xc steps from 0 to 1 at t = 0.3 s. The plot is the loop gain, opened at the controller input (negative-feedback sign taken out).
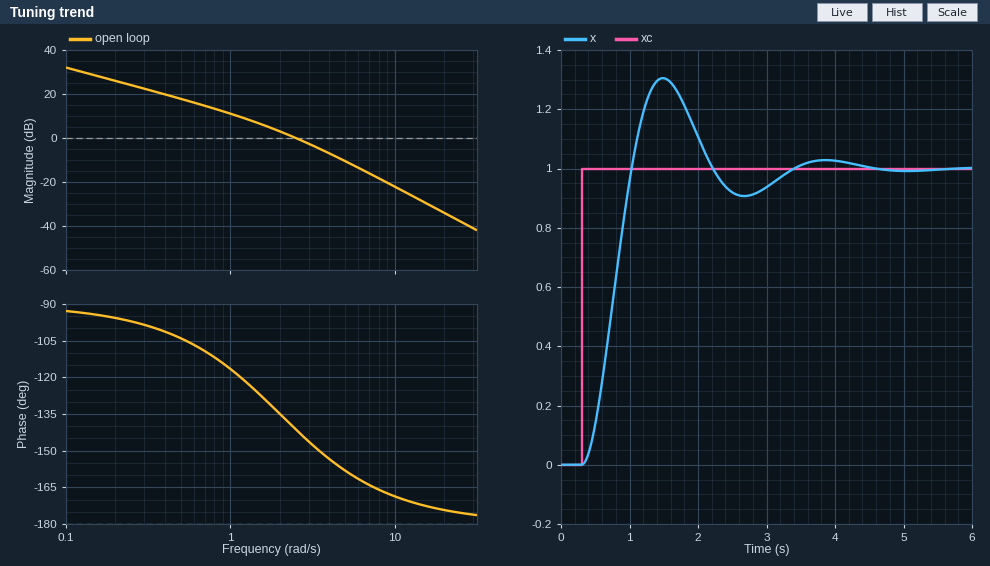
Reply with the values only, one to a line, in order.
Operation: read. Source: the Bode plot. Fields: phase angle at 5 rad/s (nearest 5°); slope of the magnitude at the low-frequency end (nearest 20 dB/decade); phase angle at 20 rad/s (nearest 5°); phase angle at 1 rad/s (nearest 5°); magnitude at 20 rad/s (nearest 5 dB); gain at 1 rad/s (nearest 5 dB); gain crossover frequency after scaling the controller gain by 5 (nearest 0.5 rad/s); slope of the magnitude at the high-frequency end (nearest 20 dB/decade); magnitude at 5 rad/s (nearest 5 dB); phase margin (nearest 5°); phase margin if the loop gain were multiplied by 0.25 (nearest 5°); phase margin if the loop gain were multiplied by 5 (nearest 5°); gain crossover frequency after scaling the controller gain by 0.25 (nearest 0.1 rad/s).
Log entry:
-160°
-20 dB/decade
-175°
-115°
-35 dB
10 dB
6.0 rad/s
-40 dB/decade
-10 dB
40°
65°
20°
0.9 rad/s
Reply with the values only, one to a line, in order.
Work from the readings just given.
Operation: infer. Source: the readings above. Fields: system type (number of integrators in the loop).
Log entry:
1
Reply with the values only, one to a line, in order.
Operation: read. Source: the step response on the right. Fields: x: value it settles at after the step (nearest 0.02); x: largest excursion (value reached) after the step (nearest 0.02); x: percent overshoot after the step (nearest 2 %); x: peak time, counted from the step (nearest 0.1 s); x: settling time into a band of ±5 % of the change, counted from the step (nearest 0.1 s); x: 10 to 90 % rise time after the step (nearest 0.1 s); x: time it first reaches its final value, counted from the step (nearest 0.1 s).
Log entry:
1.00
1.30
30 %
1.2 s
2.8 s
0.5 s
0.7 s
